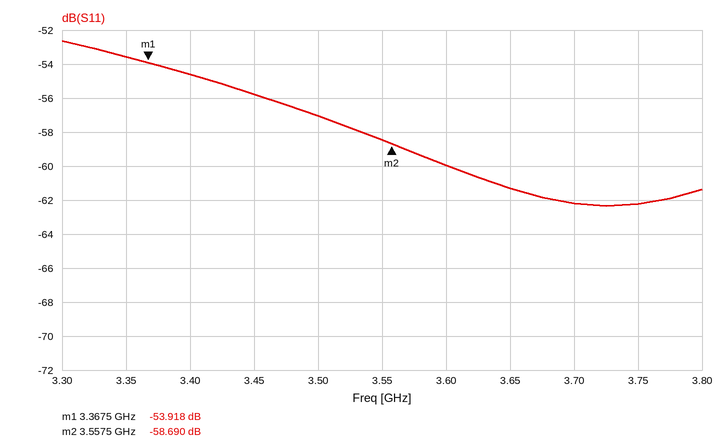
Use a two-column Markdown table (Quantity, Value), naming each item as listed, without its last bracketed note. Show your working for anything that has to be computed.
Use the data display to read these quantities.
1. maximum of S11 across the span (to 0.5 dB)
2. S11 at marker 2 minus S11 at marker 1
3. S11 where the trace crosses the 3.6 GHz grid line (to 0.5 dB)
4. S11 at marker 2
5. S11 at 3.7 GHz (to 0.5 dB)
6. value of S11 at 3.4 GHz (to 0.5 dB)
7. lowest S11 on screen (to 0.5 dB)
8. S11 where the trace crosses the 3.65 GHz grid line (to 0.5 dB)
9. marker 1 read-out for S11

| Quantity | Value |
|---|---|
| maximum of S11 across the span | -52.5 dB |
| S11 at marker 2 minus S11 at marker 1 | -58.69 − (-53.918) = -4.772 dB |
| S11 where the trace crosses the 3.6 GHz grid line | -60.0 dB |
| S11 at marker 2 | -58.690 dB |
| S11 at 3.7 GHz | -62.0 dB |
| value of S11 at 3.4 GHz | -54.5 dB |
| lowest S11 on screen | -62.5 dB |
| S11 where the trace crosses the 3.65 GHz grid line | -61.5 dB |
| marker 1 read-out for S11 | -53.918 dB |
